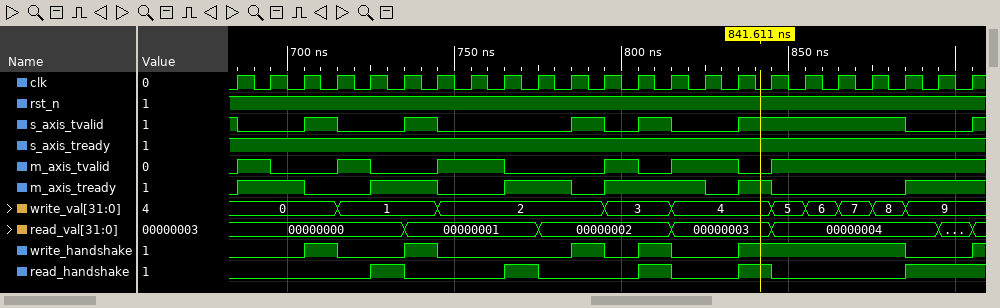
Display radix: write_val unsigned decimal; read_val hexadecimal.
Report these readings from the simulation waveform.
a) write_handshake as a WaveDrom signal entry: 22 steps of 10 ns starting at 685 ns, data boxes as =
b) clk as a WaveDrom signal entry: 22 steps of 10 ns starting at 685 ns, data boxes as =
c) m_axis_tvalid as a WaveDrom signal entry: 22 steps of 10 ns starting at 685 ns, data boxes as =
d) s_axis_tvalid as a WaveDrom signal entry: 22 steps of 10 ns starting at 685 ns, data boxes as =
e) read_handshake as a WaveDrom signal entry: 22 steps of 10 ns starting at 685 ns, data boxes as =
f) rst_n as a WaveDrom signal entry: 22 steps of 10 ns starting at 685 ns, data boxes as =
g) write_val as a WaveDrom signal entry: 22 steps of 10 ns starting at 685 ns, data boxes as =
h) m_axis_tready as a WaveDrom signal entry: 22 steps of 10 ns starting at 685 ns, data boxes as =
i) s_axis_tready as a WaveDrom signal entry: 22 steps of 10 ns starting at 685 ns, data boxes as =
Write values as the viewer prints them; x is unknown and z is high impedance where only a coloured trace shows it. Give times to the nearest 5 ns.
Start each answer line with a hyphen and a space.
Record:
- {name: 'write_handshake', wave: '0.10.10...1010.1....0.'}
- {name: 'clk', wave: 'p.....................'}
- {name: 'm_axis_tvalid', wave: '10.10.1.0..101.01.....'}
- {name: 's_axis_tvalid', wave: '0.10.10...1010.1....0.'}
- {name: 'read_handshake', wave: '0...10..10..10.10...1.'}
- {name: 'rst_n', wave: '1.....................'}
- {name: 'write_val', wave: '=..=..=....=.=..=====.', data: '0 1 2 3 4 5 6 7 8 9'}
- {name: 'm_axis_tready', wave: '1.0.1.0.1.01..010...1.'}
- {name: 's_axis_tready', wave: '1.....................'}
